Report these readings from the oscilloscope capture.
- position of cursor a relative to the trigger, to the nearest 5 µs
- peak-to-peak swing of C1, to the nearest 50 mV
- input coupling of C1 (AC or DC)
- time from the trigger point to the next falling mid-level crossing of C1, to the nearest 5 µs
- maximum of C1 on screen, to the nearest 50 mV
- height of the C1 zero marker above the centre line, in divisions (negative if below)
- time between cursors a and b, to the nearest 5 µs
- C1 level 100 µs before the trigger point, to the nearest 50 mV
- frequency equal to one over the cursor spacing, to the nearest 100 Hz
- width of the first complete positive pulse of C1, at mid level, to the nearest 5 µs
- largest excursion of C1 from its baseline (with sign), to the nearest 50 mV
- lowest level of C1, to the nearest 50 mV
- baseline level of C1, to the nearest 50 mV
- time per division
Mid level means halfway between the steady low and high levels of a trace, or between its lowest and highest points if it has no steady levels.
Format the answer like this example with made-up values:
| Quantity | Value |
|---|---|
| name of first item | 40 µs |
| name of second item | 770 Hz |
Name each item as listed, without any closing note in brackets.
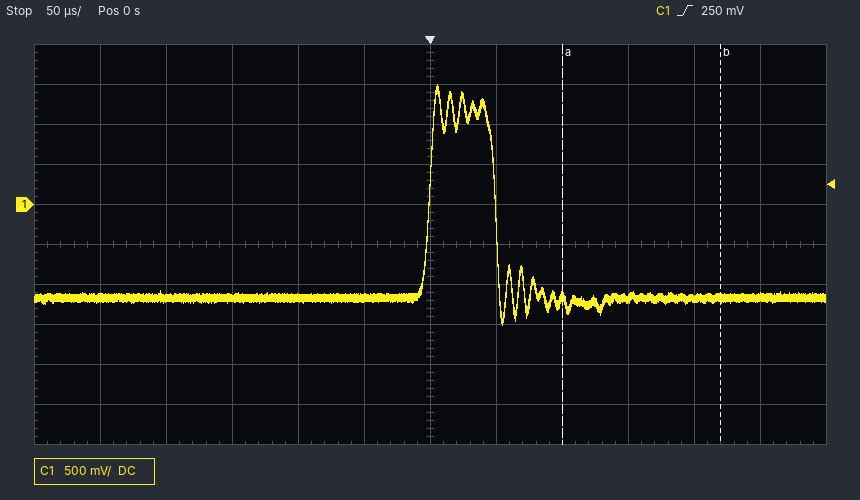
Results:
| Quantity | Value |
|---|---|
| position of cursor a relative to the trigger, to the nearest 5 µs | +100 µs |
| peak-to-peak swing of C1, to the nearest 50 mV | 3.00 V |
| input coupling of C1 | DC |
| time from the trigger point to the next falling mid-level crossing of C1, to the nearest 5 µs | 50 µs |
| maximum of C1 on screen, to the nearest 50 mV | 1.50 V |
| height of the C1 zero marker above the centre line, in divisions | +1.0 div |
| time between cursors a and b, to the nearest 5 µs | 120 µs |
| C1 level 100 µs before the trigger point, to the nearest 50 mV | -1.15 V |
| frequency equal to one over the cursor spacing, to the nearest 100 Hz | 8.3 kHz |
| width of the first complete positive pulse of C1, at mid level, to the nearest 5 µs | 50 µs |
| largest excursion of C1 from its baseline (with sign), to the nearest 50 mV | +2.65 V |
| lowest level of C1, to the nearest 50 mV | -1.50 V |
| baseline level of C1, to the nearest 50 mV | -1.15 V |
| time per division | 50 µs |
